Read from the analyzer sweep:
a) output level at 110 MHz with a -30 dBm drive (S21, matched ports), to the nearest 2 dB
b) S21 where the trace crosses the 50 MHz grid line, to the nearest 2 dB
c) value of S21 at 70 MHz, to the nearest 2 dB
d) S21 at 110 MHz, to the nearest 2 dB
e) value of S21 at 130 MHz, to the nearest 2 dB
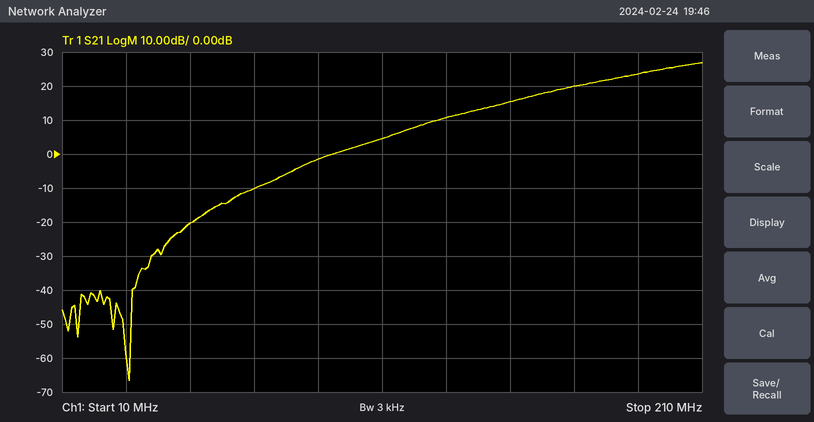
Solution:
-26 dBm
-20 dB
-10 dB
4 dB
10 dB
